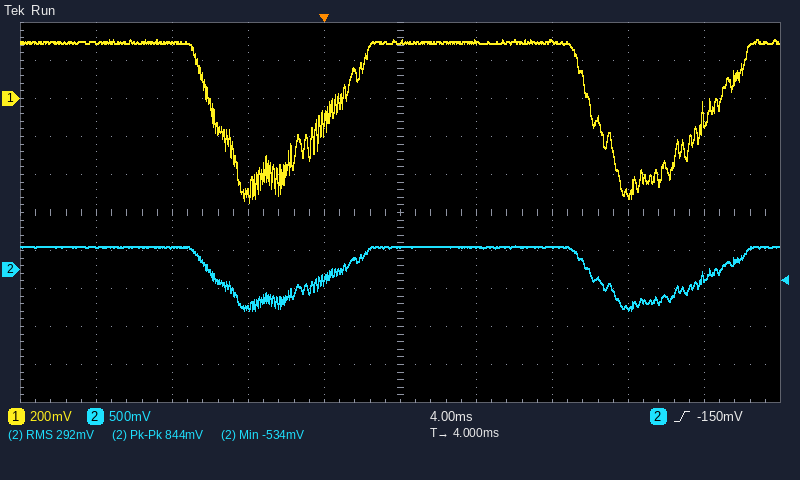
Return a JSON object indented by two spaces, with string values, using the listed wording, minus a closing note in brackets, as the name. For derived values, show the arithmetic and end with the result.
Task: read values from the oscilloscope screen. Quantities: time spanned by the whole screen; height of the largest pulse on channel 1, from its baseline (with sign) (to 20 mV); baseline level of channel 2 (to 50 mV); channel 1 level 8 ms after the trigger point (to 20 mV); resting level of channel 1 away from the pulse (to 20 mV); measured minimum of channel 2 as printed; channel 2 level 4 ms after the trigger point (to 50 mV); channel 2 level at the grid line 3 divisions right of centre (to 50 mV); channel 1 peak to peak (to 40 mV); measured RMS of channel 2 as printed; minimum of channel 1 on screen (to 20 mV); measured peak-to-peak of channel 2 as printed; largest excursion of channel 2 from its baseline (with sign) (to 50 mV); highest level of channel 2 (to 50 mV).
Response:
{
  "time spanned by the whole screen": "40 ms",
  "height of the largest pulse on channel 1, from its baseline (with sign)": "-540 mV − (300 mV) = -840 mV",
  "baseline level of channel 2": "300 mV",
  "channel 1 level 8 ms after the trigger point": "300 mV",
  "resting level of channel 1 away from the pulse": "300 mV",
  "measured minimum of channel 2 as printed": "-534 mV",
  "channel 2 level 4 ms after the trigger point": "300 mV",
  "channel 2 level at the grid line 3 divisions right of centre": "-500 mV",
  "channel 1 peak to peak": "840 mV",
  "measured RMS of channel 2 as printed": "292 mV",
  "minimum of channel 1 on screen": "-540 mV",
  "measured peak-to-peak of channel 2 as printed": "844 mV",
  "largest excursion of channel 2 from its baseline (with sign)": "-850 mV",
  "highest level of channel 2": "300 mV"
}
